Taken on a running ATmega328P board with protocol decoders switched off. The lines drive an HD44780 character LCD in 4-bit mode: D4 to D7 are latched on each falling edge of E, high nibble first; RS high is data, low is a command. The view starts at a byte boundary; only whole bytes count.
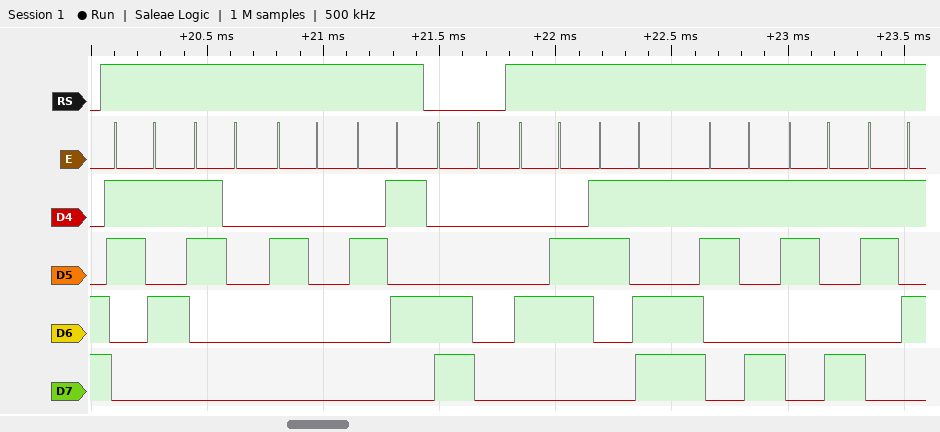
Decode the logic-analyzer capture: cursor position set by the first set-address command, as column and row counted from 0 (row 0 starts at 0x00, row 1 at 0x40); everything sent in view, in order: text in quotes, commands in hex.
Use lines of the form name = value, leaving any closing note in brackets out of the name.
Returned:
cursor position set by the first set-address command, as column and row counted from 0 = column 0, row 1
everything sent in view, in order: text in quotes, commands in hex = "50 %" 0xC0 "F=995"
